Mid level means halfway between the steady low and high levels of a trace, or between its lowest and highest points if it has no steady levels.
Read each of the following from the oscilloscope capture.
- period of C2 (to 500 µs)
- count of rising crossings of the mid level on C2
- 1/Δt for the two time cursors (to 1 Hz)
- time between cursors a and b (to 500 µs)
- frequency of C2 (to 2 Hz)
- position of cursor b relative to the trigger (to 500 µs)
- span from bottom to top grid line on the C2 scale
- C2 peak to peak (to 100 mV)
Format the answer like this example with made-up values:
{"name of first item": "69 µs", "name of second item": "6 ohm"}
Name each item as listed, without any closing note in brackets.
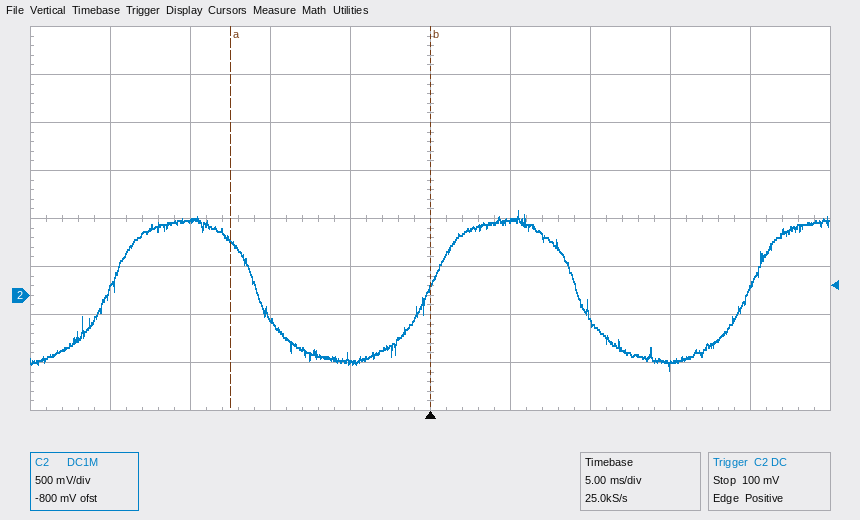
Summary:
{"period of C2": "20.0 ms", "count of rising crossings of the mid level on C2": "3", "1/Δt for the two time cursors": "80 Hz", "time between cursors a and b": "12.5 ms", "frequency of C2": "50 Hz", "position of cursor b relative to the trigger": "0.0 ms", "span from bottom to top grid line on the C2 scale": "4 V", "C2 peak to peak": "1.70 V"}
